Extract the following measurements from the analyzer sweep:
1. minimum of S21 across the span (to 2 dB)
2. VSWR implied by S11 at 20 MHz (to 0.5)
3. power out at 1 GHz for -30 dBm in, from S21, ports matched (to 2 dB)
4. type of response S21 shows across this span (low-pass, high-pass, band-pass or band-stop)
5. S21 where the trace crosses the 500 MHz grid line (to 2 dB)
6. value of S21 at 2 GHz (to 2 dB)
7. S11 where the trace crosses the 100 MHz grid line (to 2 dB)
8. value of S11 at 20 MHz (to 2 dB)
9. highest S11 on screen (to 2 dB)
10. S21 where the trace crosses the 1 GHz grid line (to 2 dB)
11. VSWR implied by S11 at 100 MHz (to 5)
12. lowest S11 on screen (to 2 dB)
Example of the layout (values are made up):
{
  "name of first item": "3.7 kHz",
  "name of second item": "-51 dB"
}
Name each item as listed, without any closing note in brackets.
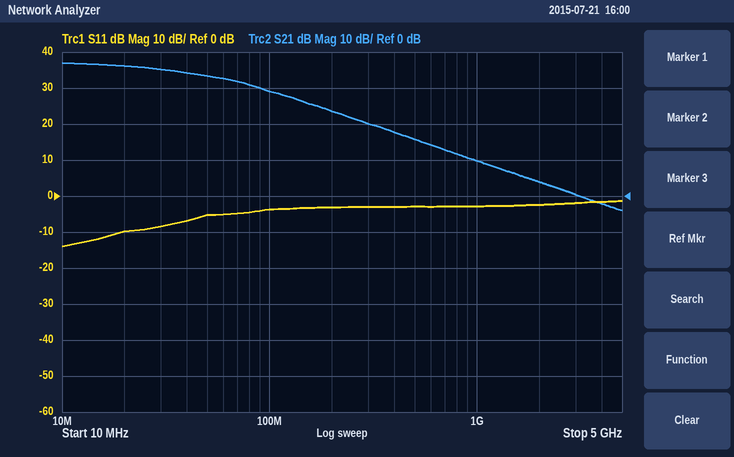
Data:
{
  "minimum of S21 across the span": "-4 dB",
  "VSWR implied by S11 at 20 MHz": "2.0",
  "power out at 1 GHz for -30 dBm in, from S21, ports matched": "-20 dBm",
  "type of response S21 shows across this span": "low-pass",
  "S21 where the trace crosses the 500 MHz grid line": "16 dB",
  "value of S21 at 2 GHz": "4 dB",
  "S11 where the trace crosses the 100 MHz grid line": "-4 dB",
  "value of S11 at 20 MHz": "-10 dB",
  "highest S11 on screen": "-2 dB",
  "S21 where the trace crosses the 1 GHz grid line": "10 dB",
  "VSWR implied by S11 at 100 MHz": "5",
  "lowest S11 on screen": "-14 dB"
}
